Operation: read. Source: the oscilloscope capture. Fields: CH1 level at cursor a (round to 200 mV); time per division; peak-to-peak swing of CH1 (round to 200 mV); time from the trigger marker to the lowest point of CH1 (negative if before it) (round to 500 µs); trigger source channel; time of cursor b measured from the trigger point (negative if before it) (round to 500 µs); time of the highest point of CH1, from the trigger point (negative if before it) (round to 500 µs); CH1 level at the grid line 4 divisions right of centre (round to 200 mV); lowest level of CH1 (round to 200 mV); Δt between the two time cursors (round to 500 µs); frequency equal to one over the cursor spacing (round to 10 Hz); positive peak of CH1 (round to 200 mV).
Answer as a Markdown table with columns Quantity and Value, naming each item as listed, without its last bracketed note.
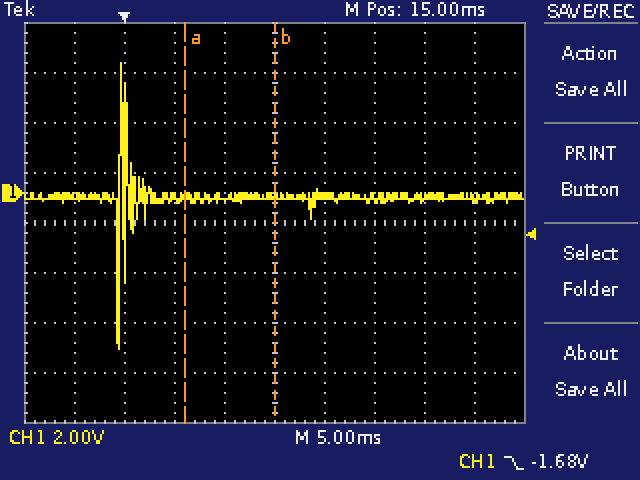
| Quantity | Value |
|---|---|
| CH1 level at cursor a | -200 mV |
| time per division | 5 ms |
| peak-to-peak swing of CH1 | 11.4 V |
| time from the trigger marker to the lowest point of CH1 (negative if before it) | -500 µs |
| trigger source channel | CH1 |
| time of cursor b measured from the trigger point (negative if before it) | +15.0 ms |
| time of the highest point of CH1, from the trigger point (negative if before it) | -500 µs |
| CH1 level at the grid line 4 divisions right of centre | -200 mV |
| lowest level of CH1 | -6.2 V |
| Δt between the two time cursors | 9.0 ms |
| frequency equal to one over the cursor spacing | 110 Hz |
| positive peak of CH1 | 5.2 V |
